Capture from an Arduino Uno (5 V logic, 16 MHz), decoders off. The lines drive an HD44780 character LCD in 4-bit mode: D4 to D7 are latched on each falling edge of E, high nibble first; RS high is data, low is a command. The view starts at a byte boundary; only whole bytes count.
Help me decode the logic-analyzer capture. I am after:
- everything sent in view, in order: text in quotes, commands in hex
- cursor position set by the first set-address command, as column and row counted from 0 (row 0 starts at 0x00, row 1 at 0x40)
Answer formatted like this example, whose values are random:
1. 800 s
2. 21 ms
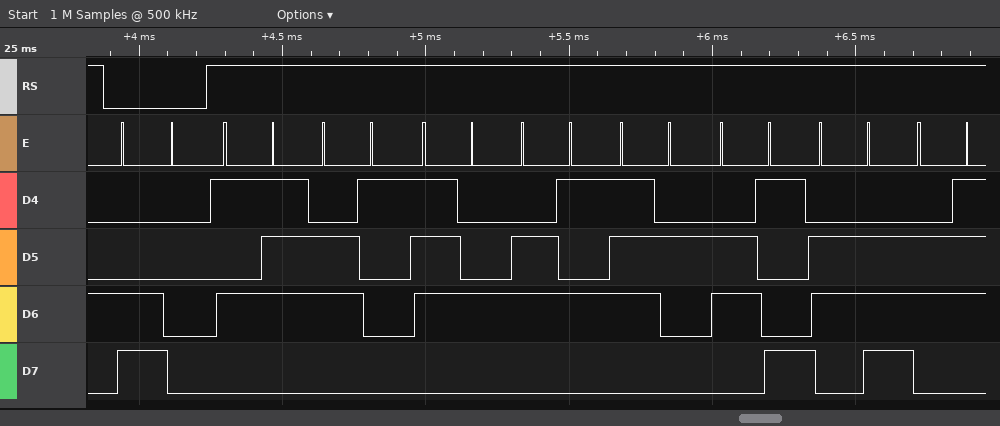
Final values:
1. 0xC0 "Watering"
2. column 0, row 1
